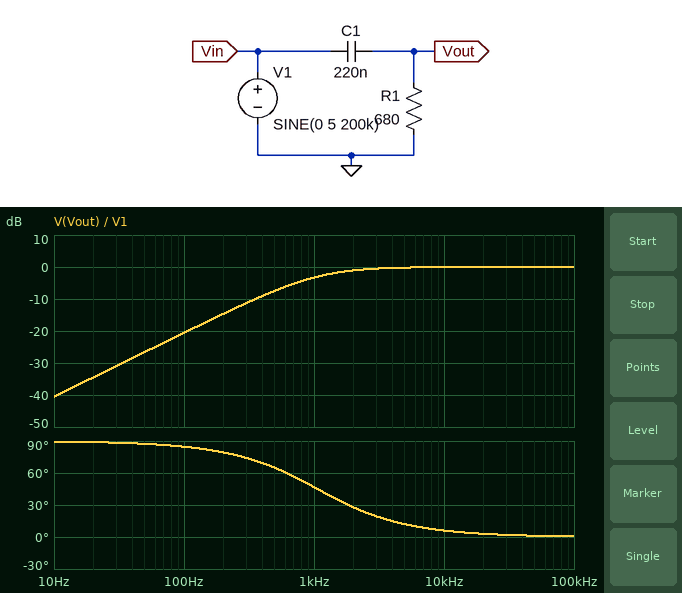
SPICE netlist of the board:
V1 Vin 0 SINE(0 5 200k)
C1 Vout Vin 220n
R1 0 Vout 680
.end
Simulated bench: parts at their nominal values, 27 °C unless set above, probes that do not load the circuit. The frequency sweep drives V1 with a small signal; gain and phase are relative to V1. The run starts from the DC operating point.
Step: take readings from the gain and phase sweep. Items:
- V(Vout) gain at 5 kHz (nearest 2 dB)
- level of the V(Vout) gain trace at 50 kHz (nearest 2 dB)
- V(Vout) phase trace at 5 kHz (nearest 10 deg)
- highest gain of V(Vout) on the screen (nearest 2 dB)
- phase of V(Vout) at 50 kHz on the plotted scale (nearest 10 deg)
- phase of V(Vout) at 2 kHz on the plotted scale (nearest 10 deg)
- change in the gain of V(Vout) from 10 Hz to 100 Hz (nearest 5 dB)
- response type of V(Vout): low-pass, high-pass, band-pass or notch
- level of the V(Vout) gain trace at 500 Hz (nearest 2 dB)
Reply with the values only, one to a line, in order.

0 dB
0 dB
10 deg
0 dB
0 deg
30 deg
20 dB
high-pass
-8 dB
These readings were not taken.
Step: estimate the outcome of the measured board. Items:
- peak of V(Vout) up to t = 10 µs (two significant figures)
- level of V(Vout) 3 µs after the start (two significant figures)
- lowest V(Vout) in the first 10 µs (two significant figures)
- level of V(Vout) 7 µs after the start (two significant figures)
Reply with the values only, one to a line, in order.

5.0 V
-3.0 V
-5.0 V
2.9 V
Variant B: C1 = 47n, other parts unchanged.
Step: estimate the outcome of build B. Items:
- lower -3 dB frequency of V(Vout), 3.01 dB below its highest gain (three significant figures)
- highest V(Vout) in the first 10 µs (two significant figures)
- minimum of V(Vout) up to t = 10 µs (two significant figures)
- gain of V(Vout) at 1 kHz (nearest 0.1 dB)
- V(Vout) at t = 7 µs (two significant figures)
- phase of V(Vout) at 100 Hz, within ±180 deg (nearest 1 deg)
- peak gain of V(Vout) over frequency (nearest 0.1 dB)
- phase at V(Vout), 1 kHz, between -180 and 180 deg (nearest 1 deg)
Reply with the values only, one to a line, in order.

4.98 kHz
4.9 V
-5.1 V
-14.1 dB
2.7 V
89 deg
0 dB
79 deg
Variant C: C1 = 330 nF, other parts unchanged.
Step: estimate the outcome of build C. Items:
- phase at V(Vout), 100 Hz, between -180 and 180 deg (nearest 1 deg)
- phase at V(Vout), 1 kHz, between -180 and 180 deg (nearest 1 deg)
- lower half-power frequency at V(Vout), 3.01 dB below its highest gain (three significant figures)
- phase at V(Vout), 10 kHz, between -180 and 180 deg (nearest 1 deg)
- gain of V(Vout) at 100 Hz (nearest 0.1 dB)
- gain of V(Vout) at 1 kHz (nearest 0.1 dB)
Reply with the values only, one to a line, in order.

82 deg
35 deg
709 Hz
4 deg
-17.1 dB
-1.8 dB
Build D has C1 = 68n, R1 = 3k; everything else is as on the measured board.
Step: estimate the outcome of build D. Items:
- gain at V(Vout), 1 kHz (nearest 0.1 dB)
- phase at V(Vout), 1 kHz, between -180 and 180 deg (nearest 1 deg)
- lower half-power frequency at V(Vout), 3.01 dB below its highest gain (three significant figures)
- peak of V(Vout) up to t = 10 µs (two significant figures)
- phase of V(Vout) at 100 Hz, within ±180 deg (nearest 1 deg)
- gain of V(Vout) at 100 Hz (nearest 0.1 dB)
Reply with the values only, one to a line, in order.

-2.1 dB
38 deg
780 Hz
5.0 V
83 deg
-17.9 dB
